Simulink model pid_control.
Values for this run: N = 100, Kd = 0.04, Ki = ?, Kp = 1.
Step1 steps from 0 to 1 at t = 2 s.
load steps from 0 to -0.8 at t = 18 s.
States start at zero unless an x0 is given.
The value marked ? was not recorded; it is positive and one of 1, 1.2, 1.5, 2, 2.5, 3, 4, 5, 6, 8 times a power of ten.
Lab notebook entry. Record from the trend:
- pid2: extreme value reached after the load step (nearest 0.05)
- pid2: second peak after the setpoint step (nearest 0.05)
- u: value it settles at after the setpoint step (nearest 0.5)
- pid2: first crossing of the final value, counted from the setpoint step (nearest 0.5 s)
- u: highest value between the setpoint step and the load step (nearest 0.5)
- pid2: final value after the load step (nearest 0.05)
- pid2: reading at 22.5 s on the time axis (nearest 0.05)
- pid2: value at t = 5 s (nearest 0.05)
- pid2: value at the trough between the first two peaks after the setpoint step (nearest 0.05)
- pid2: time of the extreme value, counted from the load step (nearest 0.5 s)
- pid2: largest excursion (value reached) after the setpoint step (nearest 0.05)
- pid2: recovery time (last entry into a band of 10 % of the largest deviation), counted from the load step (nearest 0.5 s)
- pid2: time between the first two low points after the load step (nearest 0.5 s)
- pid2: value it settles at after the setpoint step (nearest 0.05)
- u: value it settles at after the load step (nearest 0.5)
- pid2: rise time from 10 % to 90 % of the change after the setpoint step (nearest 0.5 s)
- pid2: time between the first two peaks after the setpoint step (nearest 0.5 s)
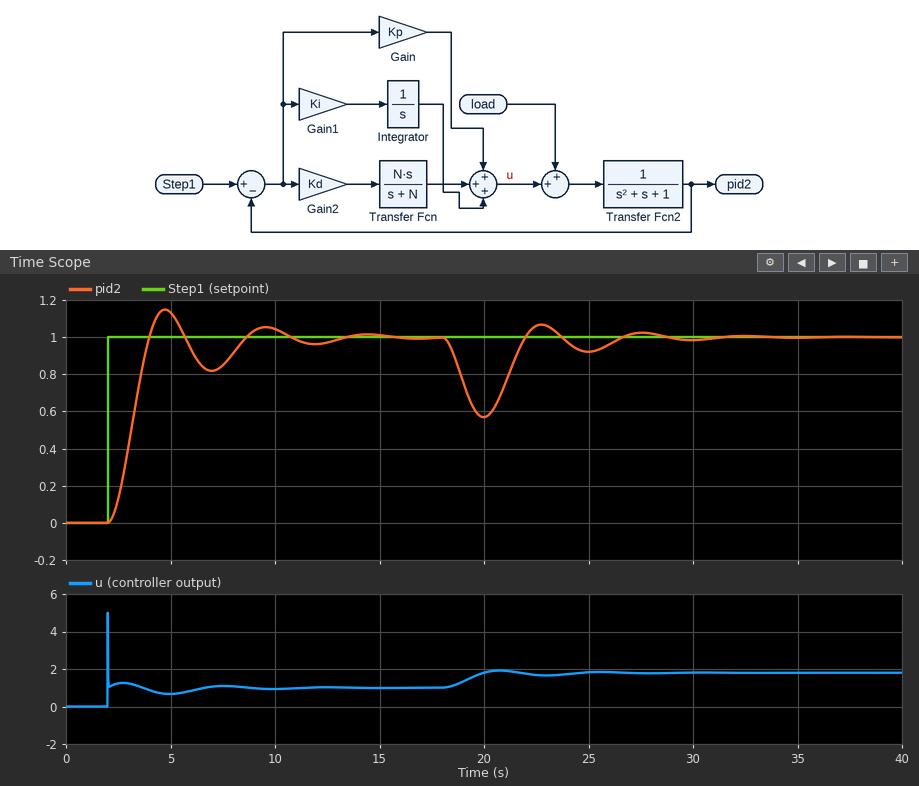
0.55
1.05
1.0
2.0 s
5.0
1.00
1.05
1.15
0.80
2.0 s
1.15
8.0 s
5.0 s
1.00
2.0
1.5 s
5.0 s
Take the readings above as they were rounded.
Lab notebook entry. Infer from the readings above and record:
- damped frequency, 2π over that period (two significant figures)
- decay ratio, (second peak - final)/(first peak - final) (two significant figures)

1.3 rad/s
0.33
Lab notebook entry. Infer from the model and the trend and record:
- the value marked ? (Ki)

0.8
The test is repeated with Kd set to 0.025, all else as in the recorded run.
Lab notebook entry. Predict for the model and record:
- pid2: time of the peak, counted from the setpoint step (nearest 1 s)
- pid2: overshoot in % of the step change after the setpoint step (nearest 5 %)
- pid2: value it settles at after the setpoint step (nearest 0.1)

3 s
15 %
1.0
